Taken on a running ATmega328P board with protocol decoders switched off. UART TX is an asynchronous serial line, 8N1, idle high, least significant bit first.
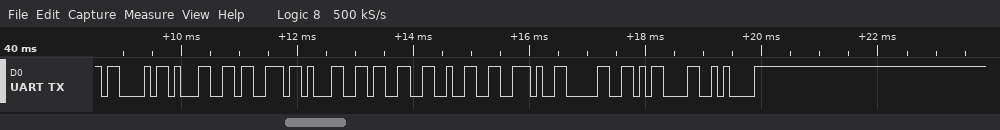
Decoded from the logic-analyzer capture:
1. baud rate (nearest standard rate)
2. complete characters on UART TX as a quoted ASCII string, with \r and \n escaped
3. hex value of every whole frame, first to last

9600 baud
"C1s132.0\r\n"
43 31 73 31 33 32 2E 30 0D 0A
